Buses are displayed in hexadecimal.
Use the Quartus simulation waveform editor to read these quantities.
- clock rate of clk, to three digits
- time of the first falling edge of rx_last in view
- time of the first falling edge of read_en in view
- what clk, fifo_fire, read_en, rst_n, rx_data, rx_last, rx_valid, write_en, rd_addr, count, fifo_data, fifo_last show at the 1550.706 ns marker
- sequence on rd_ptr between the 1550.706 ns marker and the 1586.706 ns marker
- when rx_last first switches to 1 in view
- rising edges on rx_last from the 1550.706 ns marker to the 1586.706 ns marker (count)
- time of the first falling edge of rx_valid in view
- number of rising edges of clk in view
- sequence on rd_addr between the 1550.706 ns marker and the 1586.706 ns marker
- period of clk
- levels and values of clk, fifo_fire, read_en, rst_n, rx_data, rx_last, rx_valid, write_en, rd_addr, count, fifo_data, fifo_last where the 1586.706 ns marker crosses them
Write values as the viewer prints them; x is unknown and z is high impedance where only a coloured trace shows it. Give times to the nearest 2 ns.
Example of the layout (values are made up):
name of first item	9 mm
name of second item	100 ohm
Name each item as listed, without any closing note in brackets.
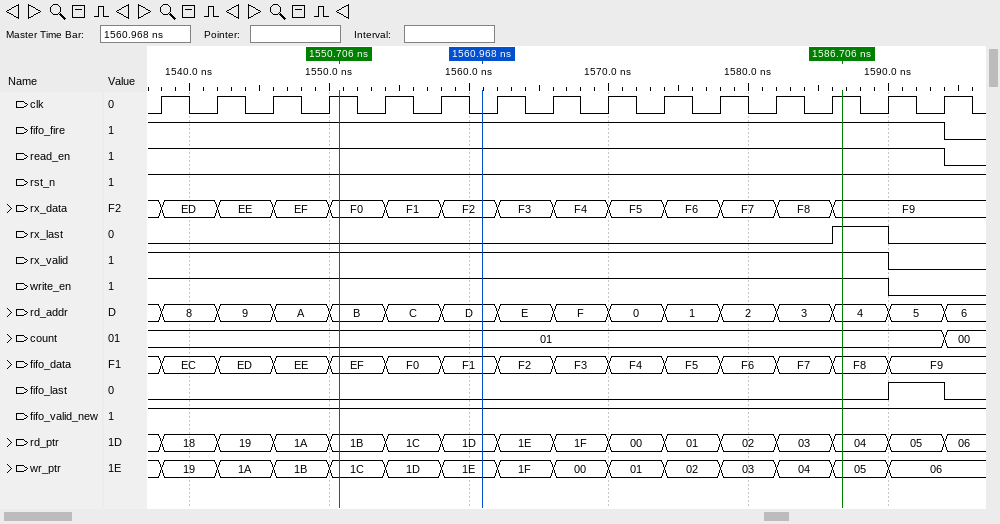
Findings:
clock rate of clk, to three digits	250 MHz
time of the first falling edge of rx_last in view	1590 ns
time of the first falling edge of read_en in view	1594 ns
what clk, fifo_fire, read_en, rst_n, rx_data, rx_last, rx_valid, write_en, rd_addr, count, fifo_data, fifo_last show at the 1550.706 ns marker	clk=1, fifo_fire=1, read_en=1, rst_n=1, rx_data=F0, rx_last=0, rx_valid=1, write_en=1, rd_addr=B, count=01, fifo_data=EF, fifo_last=0
sequence on rd_ptr between the 1550.706 ns marker and the 1586.706 ns marker	1B, 1C, 1D, 1E, 1F, 00, 01, 02, 03, 04
when rx_last first switches to 1 in view	1586 ns
rising edges on rx_last from the 1550.706 ns marker to the 1586.706 ns marker	1
time of the first falling edge of rx_valid in view	1590 ns
number of rising edges of clk in view	15
sequence on rd_addr between the 1550.706 ns marker and the 1586.706 ns marker	B, C, D, E, F, 0, 1, 2, 3, 4
period of clk	4 ns
levels and values of clk, fifo_fire, read_en, rst_n, rx_data, rx_last, rx_valid, write_en, rd_addr, count, fifo_data, fifo_last where the 1586.706 ns marker crosses them	clk=1, fifo_fire=1, read_en=1, rst_n=1, rx_data=F9, rx_last=1, rx_valid=1, write_en=1, rd_addr=4, count=01, fifo_data=F8, fifo_last=0
